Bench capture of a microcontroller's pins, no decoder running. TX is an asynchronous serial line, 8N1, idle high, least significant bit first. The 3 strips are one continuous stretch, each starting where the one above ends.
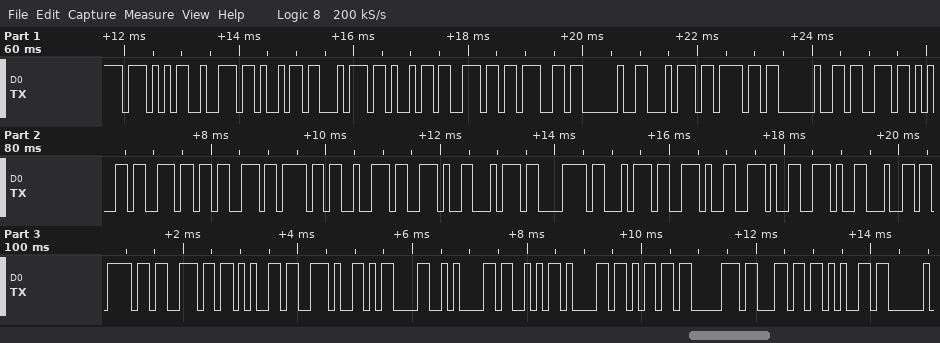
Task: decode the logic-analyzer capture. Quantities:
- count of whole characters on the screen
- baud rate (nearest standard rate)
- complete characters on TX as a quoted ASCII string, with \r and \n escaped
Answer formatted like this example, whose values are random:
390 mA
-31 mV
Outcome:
37
9600 baud
"Writing to sensor.txt...done.\r\nSample"
